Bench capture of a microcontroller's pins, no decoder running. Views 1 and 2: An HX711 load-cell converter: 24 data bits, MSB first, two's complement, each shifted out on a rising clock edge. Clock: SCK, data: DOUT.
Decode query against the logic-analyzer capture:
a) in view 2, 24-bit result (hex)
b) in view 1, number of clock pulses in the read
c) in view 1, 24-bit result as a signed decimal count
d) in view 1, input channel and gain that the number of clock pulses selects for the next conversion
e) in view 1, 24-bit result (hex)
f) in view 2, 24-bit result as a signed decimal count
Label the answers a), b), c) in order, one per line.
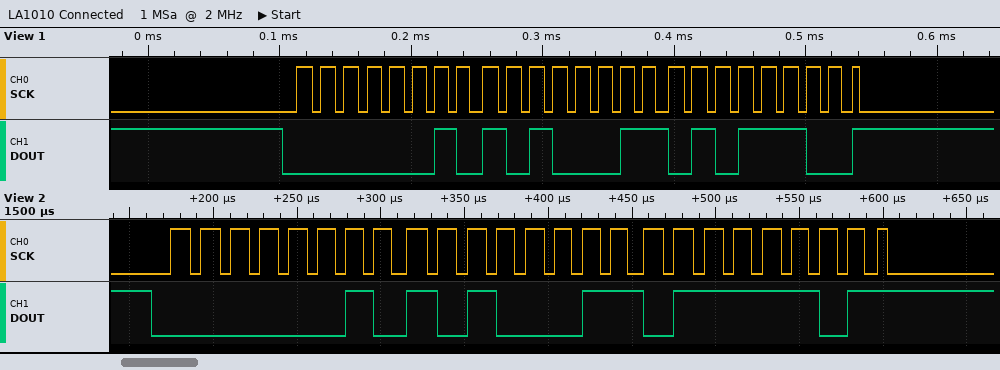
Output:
a) 0x02A37D
b) 25
c) 172892
d) channel A, gain 128
e) 0x02A35C
f) 172925
